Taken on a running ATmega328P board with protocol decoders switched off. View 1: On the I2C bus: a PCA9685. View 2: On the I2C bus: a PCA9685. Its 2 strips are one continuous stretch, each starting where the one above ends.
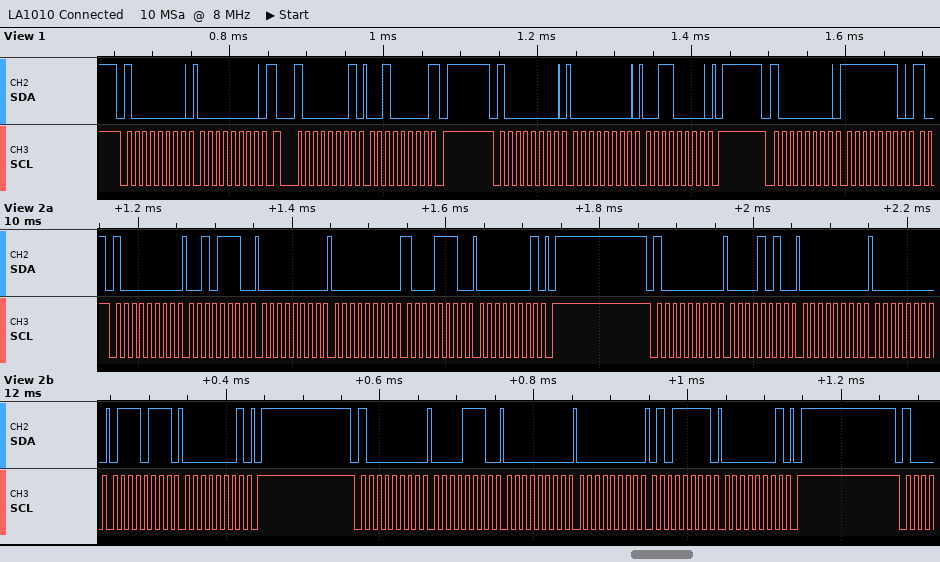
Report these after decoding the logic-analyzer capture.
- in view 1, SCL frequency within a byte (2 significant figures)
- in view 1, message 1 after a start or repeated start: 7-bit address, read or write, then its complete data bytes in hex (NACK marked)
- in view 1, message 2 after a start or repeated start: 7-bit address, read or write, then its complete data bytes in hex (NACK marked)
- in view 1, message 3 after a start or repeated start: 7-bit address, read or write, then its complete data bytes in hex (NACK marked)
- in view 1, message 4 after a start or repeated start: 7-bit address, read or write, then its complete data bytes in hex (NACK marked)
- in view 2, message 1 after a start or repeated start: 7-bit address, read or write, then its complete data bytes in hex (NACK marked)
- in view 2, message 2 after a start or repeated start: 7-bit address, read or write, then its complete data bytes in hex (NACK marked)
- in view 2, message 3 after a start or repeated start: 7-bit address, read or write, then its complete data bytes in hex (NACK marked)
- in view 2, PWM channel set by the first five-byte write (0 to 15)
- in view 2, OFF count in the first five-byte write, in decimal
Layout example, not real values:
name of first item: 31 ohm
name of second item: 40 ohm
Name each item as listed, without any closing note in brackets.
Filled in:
in view 1, SCL frequency within a byte: 100 kHz
in view 1, message 1 after a start or repeated start: 7-bit address, read or write, then its complete data bytes in hex: 0x40 write: 00
in view 1, message 2 after a start or repeated start: 7-bit address, read or write, then its complete data bytes in hex: 0x40 read: 20 NACK
in view 1, message 3 after a start or repeated start: 7-bit address, read or write, then its complete data bytes in hex: 0x40 write: 00 30
in view 1, message 4 after a start or repeated start: 7-bit address, read or write, then its complete data bytes in hex: 0x40 write: FE
in view 2, message 1 after a start or repeated start: 7-bit address, read or write, then its complete data bytes in hex: 0x40 write: 2E 00 00 8E 01
in view 2, message 2 after a start or repeated start: 7-bit address, read or write, then its complete data bytes in hex: 0x40 write: 0A 00 00 77 01
in view 2, message 3 after a start or repeated start: 7-bit address, read or write, then its complete data bytes in hex: 0x40 write: 0E 00 00 5F 01
in view 2, PWM channel set by the first five-byte write: 10
in view 2, OFF count in the first five-byte write, in decimal: 398
